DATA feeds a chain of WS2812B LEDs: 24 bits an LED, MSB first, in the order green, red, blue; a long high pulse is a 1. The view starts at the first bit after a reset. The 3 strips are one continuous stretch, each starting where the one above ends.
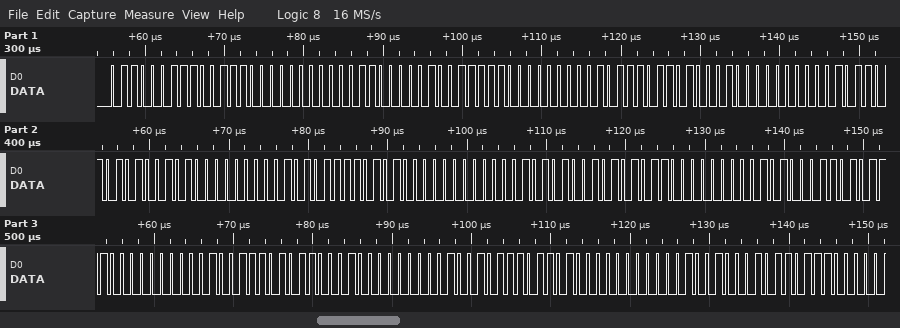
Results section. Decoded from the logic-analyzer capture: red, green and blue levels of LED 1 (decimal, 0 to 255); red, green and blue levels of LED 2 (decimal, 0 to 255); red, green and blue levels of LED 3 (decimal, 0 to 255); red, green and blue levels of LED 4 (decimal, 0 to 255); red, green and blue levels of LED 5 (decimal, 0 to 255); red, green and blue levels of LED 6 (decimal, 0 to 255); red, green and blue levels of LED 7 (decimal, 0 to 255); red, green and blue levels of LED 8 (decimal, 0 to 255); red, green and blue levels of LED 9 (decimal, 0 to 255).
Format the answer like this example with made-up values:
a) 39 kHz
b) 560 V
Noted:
a) 156, 99, 0
b) 159, 96, 0
c) 162, 93, 0
d) 165, 90, 0
e) 168, 87, 0
f) 171, 84, 0
g) 174, 81, 0
h) 177, 78, 0
i) 180, 75, 0
